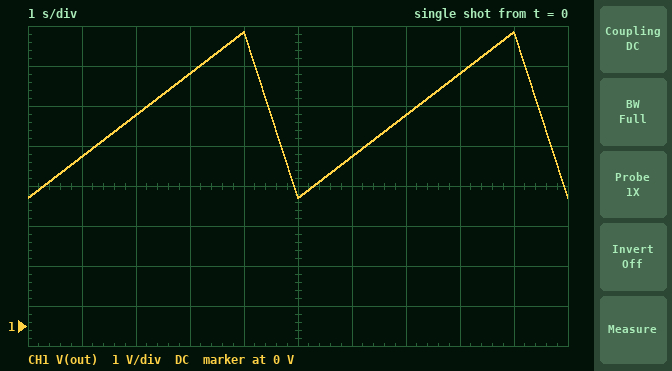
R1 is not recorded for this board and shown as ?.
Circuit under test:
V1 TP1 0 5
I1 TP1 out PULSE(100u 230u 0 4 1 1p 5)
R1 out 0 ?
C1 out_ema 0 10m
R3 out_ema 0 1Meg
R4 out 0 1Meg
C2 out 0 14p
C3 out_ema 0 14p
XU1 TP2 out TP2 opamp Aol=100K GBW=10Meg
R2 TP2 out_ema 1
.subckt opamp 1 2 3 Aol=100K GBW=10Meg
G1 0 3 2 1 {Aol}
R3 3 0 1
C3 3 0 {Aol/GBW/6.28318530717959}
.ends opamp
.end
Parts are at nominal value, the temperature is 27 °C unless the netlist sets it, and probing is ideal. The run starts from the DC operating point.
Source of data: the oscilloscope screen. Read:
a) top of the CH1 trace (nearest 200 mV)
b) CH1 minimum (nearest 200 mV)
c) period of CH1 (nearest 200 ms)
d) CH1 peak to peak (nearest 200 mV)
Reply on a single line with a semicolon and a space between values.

7.4 V; 3.2 V; 5.0 s; 4.2 V
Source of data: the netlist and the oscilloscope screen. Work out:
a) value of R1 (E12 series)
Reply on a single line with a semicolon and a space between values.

33 kΩ
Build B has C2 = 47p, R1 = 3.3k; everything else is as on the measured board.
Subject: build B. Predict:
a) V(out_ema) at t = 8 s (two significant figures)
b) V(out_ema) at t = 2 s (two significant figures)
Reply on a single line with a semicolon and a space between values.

650 mV; 540 mV
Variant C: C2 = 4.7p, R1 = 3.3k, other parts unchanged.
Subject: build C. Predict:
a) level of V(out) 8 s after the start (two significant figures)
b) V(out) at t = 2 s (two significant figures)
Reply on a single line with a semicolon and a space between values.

650 mV; 540 mV
